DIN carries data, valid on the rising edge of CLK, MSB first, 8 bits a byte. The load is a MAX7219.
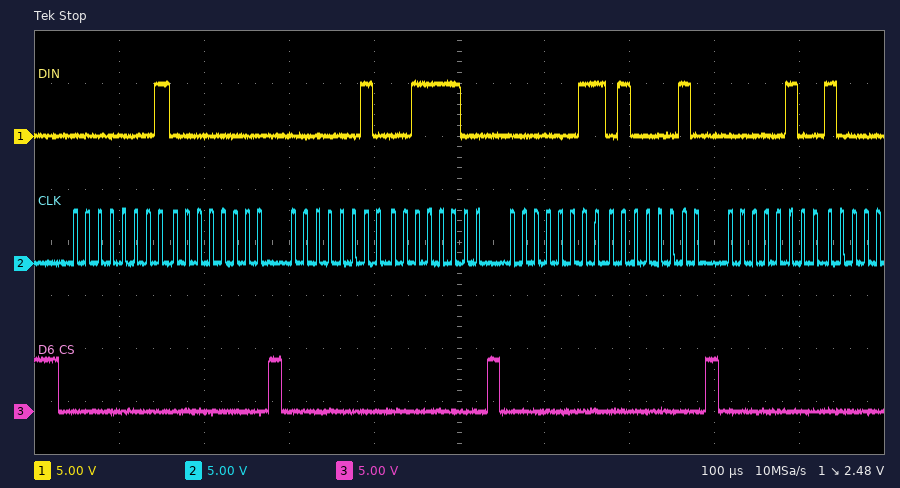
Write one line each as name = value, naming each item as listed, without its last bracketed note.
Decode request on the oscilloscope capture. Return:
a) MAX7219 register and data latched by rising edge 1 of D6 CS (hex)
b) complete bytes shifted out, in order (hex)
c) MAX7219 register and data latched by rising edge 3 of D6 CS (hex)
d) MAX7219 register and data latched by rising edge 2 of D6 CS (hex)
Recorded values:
MAX7219 register and data latched by rising edge 1 of D6 CS = register 0x1, data 0x00
complete bytes shifted out, in order = 0x01 0x00 0x02 0x3C 0x03 0x42 0x04
MAX7219 register and data latched by rising edge 3 of D6 CS = register 0x3, data 0x42
MAX7219 register and data latched by rising edge 2 of D6 CS = register 0x2, data 0x3C
